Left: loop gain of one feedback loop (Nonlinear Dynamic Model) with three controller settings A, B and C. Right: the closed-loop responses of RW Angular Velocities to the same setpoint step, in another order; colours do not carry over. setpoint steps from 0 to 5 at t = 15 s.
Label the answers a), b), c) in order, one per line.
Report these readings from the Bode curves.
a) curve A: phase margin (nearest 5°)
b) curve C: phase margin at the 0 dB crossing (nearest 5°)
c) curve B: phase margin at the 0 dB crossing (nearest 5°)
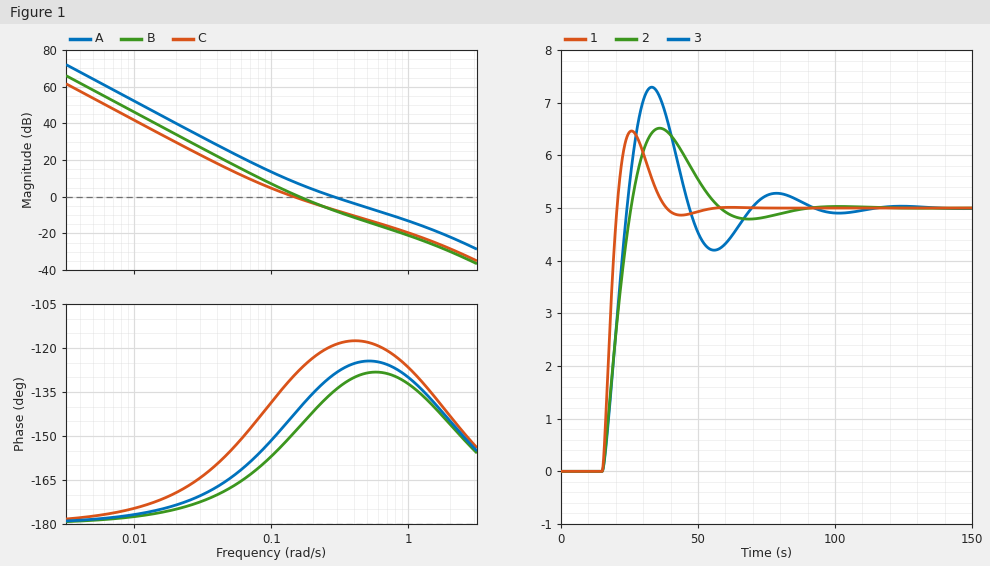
a) 50°
b) 50°
c) 35°
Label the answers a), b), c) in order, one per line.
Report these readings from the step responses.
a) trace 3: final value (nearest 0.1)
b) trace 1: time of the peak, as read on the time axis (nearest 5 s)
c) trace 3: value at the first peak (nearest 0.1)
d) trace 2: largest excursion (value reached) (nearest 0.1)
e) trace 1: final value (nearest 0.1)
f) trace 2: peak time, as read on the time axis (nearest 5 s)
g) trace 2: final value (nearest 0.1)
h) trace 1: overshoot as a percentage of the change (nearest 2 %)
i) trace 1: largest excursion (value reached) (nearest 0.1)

a) 5.0
b) 25 s
c) 7.3
d) 6.5
e) 5.0
f) 35 s
g) 5.0
h) 30 %
i) 6.5
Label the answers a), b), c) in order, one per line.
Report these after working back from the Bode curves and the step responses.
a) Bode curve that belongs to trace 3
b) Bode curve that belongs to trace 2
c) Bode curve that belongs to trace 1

a) B
b) C
c) A
